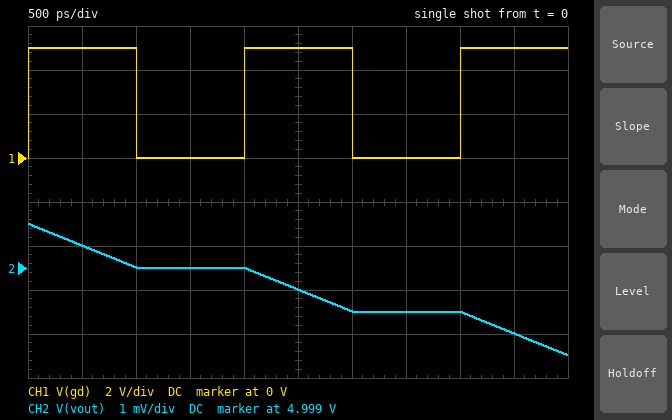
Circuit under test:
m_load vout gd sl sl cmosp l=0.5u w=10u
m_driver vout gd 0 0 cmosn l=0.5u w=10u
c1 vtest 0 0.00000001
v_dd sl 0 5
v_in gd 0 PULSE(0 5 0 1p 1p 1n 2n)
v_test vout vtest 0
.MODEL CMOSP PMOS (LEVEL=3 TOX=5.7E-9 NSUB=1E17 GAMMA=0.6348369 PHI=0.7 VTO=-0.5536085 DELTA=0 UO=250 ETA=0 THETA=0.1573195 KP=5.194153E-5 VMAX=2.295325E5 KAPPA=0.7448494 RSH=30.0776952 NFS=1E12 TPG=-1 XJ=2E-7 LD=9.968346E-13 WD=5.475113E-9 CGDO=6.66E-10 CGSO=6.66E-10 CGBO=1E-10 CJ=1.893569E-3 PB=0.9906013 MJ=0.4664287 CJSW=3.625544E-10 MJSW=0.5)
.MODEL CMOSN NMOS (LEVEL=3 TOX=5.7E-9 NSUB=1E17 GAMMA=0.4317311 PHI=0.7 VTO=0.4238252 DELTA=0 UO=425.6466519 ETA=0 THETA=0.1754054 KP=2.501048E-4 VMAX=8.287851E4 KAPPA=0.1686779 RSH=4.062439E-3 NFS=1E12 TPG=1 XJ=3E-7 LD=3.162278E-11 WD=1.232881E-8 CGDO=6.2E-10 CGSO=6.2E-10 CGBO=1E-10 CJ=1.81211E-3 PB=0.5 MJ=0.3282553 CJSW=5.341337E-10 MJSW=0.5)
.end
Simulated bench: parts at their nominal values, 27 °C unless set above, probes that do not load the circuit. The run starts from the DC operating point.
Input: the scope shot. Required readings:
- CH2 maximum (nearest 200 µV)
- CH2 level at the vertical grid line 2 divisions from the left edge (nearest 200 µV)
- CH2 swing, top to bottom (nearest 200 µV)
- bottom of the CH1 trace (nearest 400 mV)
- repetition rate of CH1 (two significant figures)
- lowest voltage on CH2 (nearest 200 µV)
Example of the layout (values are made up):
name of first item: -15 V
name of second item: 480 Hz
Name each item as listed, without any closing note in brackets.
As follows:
CH2 maximum: 5.0000 V
CH2 level at the vertical grid line 2 divisions from the left edge: 4.9990 V
CH2 swing, top to bottom: 3.0 mV
bottom of the CH1 trace: 0 V
repetition rate of CH1: 500 MHz
lowest voltage on CH2: 4.9970 V
